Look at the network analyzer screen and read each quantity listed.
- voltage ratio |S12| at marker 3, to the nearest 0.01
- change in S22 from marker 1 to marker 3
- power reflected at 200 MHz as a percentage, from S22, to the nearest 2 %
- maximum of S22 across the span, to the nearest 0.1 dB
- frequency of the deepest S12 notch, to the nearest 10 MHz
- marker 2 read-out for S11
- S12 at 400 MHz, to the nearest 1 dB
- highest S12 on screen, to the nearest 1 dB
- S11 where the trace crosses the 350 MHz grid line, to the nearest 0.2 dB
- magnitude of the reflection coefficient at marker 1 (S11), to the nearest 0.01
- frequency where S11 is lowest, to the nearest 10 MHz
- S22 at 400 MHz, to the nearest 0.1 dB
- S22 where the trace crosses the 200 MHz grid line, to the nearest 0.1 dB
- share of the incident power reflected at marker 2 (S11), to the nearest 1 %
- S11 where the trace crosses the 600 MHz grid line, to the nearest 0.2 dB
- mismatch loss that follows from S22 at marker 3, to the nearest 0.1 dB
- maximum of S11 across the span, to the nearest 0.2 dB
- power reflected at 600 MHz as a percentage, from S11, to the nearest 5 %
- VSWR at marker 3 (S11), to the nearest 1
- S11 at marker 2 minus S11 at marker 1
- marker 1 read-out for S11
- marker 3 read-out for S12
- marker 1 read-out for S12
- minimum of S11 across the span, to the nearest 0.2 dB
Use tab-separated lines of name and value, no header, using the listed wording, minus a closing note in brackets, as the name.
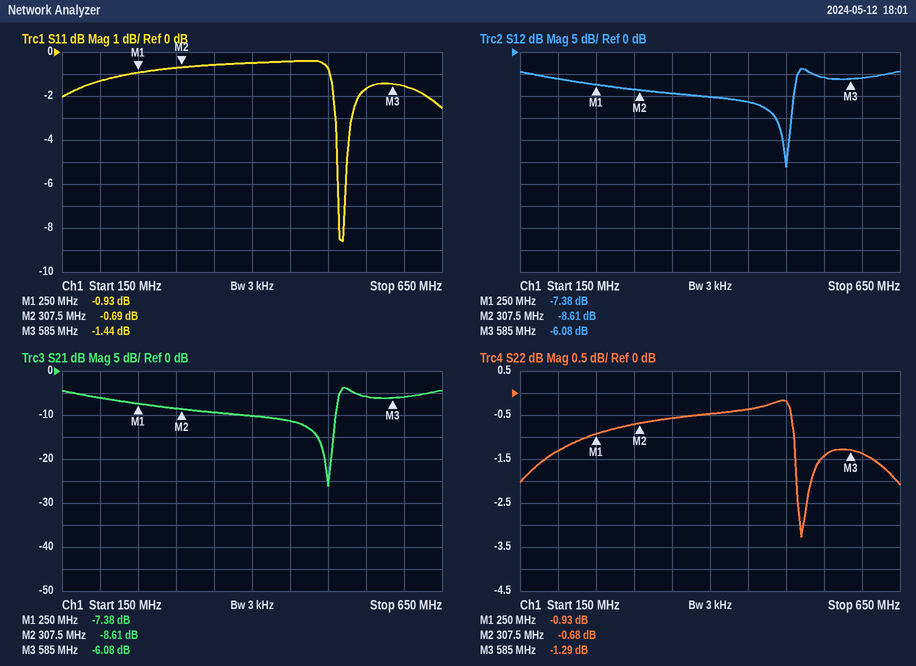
voltage ratio |S12| at marker 3, to the nearest 0.01	0.50
change in S22 from marker 1 to marker 3	-0.36 dB
power reflected at 200 MHz as a percentage, from S22, to the nearest 2 %	74 %
maximum of S22 across the span, to the nearest 0.1 dB	-0.2 dB
frequency of the deepest S12 notch, to the nearest 10 MHz	500 MHz
marker 2 read-out for S11	-0.69 dB
S12 at 400 MHz, to the nearest 1 dB	-10 dB
highest S12 on screen, to the nearest 1 dB	-4 dB
S11 where the trace crosses the 350 MHz grid line, to the nearest 0.2 dB	-0.6 dB
magnitude of the reflection coefficient at marker 1 (S11), to the nearest 0.01	0.90
frequency where S11 is lowest, to the nearest 10 MHz	520 MHz
S22 at 400 MHz, to the nearest 0.1 dB	-0.5 dB
S22 where the trace crosses the 200 MHz grid line, to the nearest 0.1 dB	-1.3 dB
share of the incident power reflected at marker 2 (S11), to the nearest 1 %	85 %
S11 where the trace crosses the 600 MHz grid line, to the nearest 0.2 dB	-1.6 dB
mismatch loss that follows from S22 at marker 3, to the nearest 0.1 dB	5.9 dB
maximum of S11 across the span, to the nearest 0.2 dB	-0.4 dB
power reflected at 600 MHz as a percentage, from S11, to the nearest 5 %	70 %
VSWR at marker 3 (S11), to the nearest 1	12
S11 at marker 2 minus S11 at marker 1	0.24 dB
marker 1 read-out for S11	-0.93 dB
marker 3 read-out for S12	-6.08 dB
marker 1 read-out for S12	-7.38 dB
minimum of S11 across the span, to the nearest 0.2 dB	-8.6 dB
